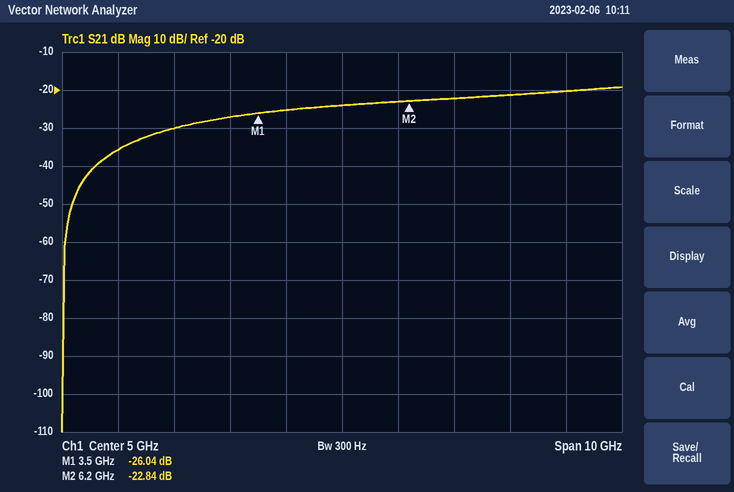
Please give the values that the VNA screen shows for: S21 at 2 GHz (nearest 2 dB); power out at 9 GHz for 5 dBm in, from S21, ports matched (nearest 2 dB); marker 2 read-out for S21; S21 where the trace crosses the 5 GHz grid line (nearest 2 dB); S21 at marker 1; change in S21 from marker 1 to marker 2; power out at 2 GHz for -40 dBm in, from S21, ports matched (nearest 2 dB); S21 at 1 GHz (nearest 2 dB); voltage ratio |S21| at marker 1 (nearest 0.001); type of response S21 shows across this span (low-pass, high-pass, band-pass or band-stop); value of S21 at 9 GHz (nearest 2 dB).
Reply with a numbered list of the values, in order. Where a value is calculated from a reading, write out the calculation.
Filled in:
1. -30 dB
2. 5 dBm + (-20 dB) = -16 dBm
3. -22.84 dB
4. -24 dB
5. -26.04 dB
6. -22.84 − (-26.04) = 3.20 dB
7. -40 dBm + (-30 dB) = -70 dBm
8. -36 dB
9. 10^(-26.04/20) ≈ 0.050
10. high-pass
11. -20 dB
